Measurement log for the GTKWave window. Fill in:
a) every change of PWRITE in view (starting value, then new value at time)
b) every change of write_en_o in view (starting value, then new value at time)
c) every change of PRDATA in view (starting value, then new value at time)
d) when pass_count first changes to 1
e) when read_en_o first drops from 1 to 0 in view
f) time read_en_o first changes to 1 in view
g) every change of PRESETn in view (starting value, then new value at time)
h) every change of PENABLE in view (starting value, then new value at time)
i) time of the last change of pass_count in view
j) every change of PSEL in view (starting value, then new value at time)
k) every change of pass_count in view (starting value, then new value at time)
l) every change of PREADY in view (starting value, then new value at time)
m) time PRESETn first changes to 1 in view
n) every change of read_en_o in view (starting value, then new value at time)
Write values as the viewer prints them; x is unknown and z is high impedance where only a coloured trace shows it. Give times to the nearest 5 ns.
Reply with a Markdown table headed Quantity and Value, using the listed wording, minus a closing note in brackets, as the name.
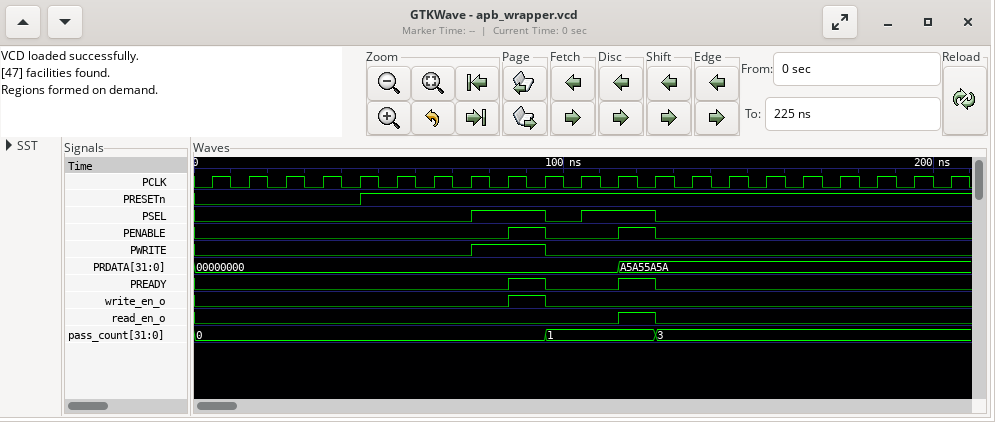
| Quantity | Value |
|---|---|
| every change of PWRITE in view | 0, 1 at 75 ns, 0 at 95 ns |
| every change of write_en_o in view | 0, 1 at 85 ns, 0 at 95 ns |
| every change of PRDATA in view | 00000000, A5A55A5A at 115 ns |
| when pass_count first changes to 1 | 95 ns |
| when read_en_o first drops from 1 to 0 in view | 125 ns |
| time read_en_o first changes to 1 in view | 115 ns |
| every change of PRESETn in view | 0, 1 at 45 ns |
| every change of PENABLE in view | 0, 1 at 85 ns, 0 at 95 ns, 1 at 115 ns, 0 at 125 ns |
| time of the last change of pass_count in view | 125 ns |
| every change of PSEL in view | 0, 1 at 75 ns, 0 at 95 ns, 1 at 105 ns, 0 at 125 ns |
| every change of pass_count in view | 0, 1 at 95 ns, 3 at 125 ns |
| every change of PREADY in view | 0, 1 at 85 ns, 0 at 95 ns, 1 at 115 ns, 0 at 125 ns |
| time PRESETn first changes to 1 in view | 45 ns |
| every change of read_en_o in view | 0, 1 at 115 ns, 0 at 125 ns |
